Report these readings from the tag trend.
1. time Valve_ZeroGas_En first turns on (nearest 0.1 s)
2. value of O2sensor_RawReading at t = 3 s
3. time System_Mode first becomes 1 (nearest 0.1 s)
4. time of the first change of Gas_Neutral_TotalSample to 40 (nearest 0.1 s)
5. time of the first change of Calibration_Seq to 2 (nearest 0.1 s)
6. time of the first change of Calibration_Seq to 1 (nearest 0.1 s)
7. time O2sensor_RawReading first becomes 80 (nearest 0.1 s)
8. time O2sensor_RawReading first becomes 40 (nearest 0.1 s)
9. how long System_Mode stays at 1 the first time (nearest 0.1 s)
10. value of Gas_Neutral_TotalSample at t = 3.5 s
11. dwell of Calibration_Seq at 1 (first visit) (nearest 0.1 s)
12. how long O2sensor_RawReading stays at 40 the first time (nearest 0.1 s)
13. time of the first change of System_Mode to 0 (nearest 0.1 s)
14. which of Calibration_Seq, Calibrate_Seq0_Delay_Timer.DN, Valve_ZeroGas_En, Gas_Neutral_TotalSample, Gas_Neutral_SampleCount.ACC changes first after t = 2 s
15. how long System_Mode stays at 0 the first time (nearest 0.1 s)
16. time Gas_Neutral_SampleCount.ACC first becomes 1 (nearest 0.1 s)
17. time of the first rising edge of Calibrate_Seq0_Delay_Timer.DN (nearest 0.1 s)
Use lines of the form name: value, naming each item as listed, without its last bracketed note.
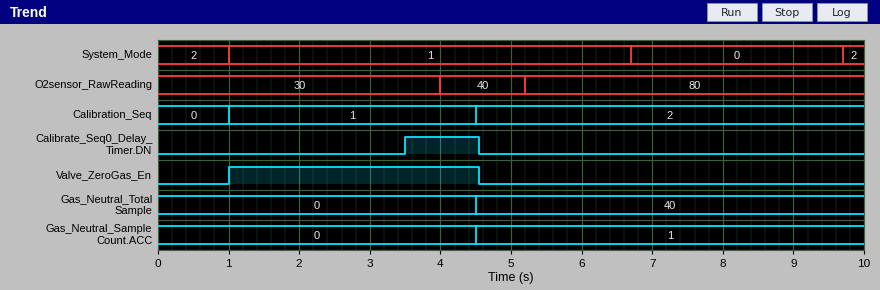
time Valve_ZeroGas_En first turns on: 1.0 s
value of O2sensor_RawReading at t = 3 s: 30
time System_Mode first becomes 1: 1.0 s
time of the first change of Gas_Neutral_TotalSample to 40: 4.5 s
time of the first change of Calibration_Seq to 2: 4.5 s
time of the first change of Calibration_Seq to 1: 1.0 s
time O2sensor_RawReading first becomes 80: 5.2 s
time O2sensor_RawReading first becomes 40: 4.0 s
how long System_Mode stays at 1 the first time: 5.7 s
value of Gas_Neutral_TotalSample at t = 3.5 s: 0
dwell of Calibration_Seq at 1 (first visit): 3.5 s
how long O2sensor_RawReading stays at 40 the first time: 1.2 s
time of the first change of System_Mode to 0: 6.7 s
which of Calibration_Seq, Calibrate_Seq0_Delay_Timer.DN, Valve_ZeroGas_En, Gas_Neutral_TotalSample, Gas_Neutral_SampleCount.ACC changes first after t = 2 s: Calibrate_Seq0_Delay_Timer.DN
how long System_Mode stays at 0 the first time: 3.0 s
time Gas_Neutral_SampleCount.ACC first becomes 1: 4.5 s
time of the first rising edge of Calibrate_Seq0_Delay_Timer.DN: 3.5 s
